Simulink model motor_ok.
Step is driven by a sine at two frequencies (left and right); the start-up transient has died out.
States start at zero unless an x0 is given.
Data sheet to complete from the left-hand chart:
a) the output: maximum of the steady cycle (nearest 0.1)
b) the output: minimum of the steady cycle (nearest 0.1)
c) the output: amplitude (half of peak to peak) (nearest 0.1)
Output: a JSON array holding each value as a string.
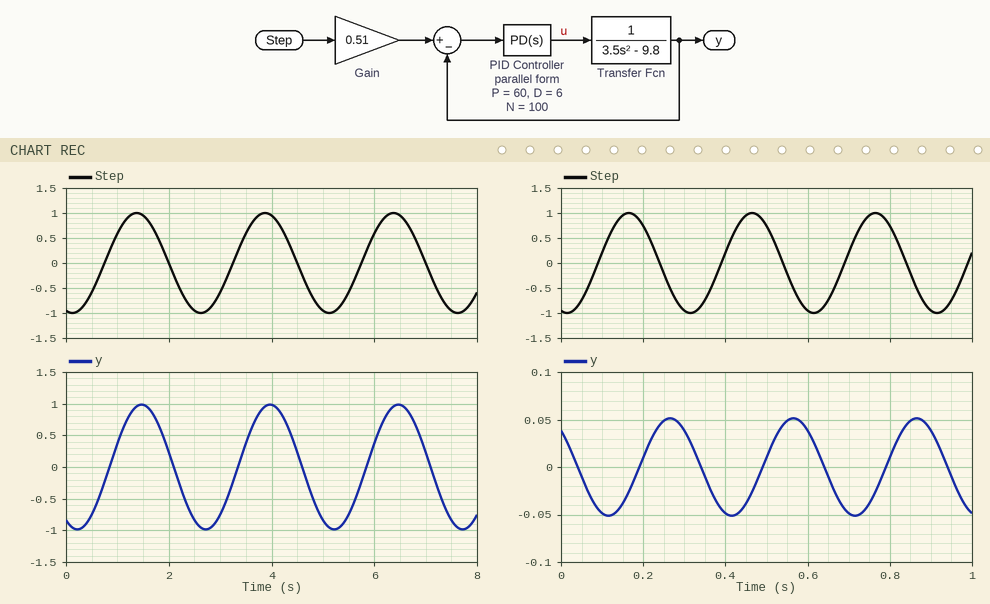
["1.0", "-1.0", "1.0"]
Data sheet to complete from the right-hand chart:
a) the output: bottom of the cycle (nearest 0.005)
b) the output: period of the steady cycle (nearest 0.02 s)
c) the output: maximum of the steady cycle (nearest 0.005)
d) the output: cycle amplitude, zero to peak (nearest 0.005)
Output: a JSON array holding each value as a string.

["-0.050", "0.30 s", "0.050", "0.050"]
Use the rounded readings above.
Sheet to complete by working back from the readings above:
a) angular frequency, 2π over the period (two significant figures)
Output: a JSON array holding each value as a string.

["21 rad/s"]
